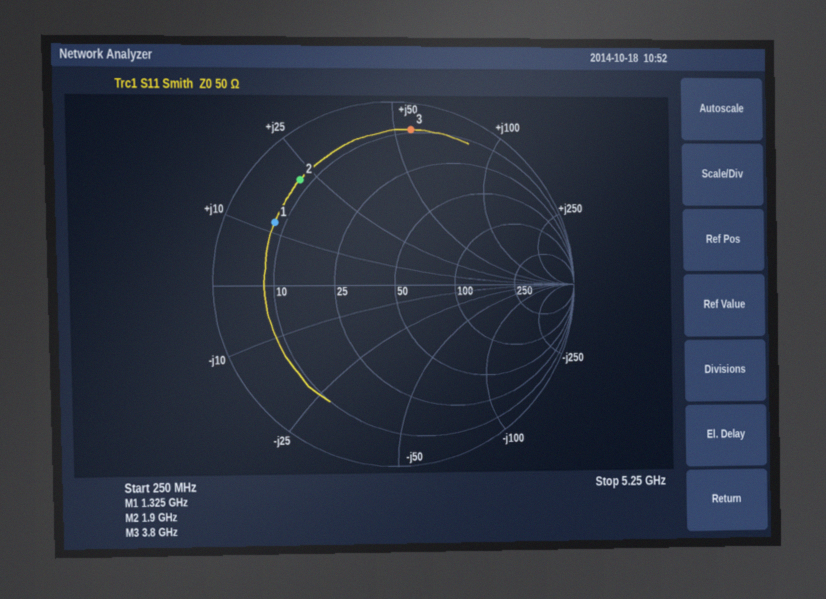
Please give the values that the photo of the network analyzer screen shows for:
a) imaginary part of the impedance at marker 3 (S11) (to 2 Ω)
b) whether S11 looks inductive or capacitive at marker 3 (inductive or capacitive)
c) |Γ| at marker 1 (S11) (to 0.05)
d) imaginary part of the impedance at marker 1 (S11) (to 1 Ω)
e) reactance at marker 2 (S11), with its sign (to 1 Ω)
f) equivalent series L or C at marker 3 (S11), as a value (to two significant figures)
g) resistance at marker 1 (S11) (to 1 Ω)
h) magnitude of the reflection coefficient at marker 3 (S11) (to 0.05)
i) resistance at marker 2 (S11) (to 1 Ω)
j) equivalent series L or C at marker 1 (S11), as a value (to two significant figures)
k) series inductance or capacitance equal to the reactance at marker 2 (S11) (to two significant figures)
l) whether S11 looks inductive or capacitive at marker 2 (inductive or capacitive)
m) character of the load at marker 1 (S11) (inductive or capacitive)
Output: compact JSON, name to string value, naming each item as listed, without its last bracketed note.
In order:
{"imaginary part of the impedance at marker 3 (S11)": "+56 Ω", "whether S11 looks inductive or capacitive at marker 3": "inductive", "|Γ| at marker 1 (S11)": "0.75", "imaginary part of the impedance at marker 1 (S11)": "+12 Ω", "reactance at marker 2 (S11), with its sign": "+22 Ω", "equivalent series L or C at marker 3 (S11), as a value": "2.3 nH", "resistance at marker 1 (S11)": "8 Ω", "magnitude of the reflection coefficient at marker 3 (S11)": "0.85", "resistance at marker 2 (S11)": "8 Ω", "equivalent series L or C at marker 1 (S11), as a value": "1.4 nH", "series inductance or capacitance equal to the reactance at marker 2 (S11)": "1.8 nH", "whether S11 looks inductive or capacitive at marker 2": "inductive", "character of the load at marker 1 (S11)": "inductive"}
